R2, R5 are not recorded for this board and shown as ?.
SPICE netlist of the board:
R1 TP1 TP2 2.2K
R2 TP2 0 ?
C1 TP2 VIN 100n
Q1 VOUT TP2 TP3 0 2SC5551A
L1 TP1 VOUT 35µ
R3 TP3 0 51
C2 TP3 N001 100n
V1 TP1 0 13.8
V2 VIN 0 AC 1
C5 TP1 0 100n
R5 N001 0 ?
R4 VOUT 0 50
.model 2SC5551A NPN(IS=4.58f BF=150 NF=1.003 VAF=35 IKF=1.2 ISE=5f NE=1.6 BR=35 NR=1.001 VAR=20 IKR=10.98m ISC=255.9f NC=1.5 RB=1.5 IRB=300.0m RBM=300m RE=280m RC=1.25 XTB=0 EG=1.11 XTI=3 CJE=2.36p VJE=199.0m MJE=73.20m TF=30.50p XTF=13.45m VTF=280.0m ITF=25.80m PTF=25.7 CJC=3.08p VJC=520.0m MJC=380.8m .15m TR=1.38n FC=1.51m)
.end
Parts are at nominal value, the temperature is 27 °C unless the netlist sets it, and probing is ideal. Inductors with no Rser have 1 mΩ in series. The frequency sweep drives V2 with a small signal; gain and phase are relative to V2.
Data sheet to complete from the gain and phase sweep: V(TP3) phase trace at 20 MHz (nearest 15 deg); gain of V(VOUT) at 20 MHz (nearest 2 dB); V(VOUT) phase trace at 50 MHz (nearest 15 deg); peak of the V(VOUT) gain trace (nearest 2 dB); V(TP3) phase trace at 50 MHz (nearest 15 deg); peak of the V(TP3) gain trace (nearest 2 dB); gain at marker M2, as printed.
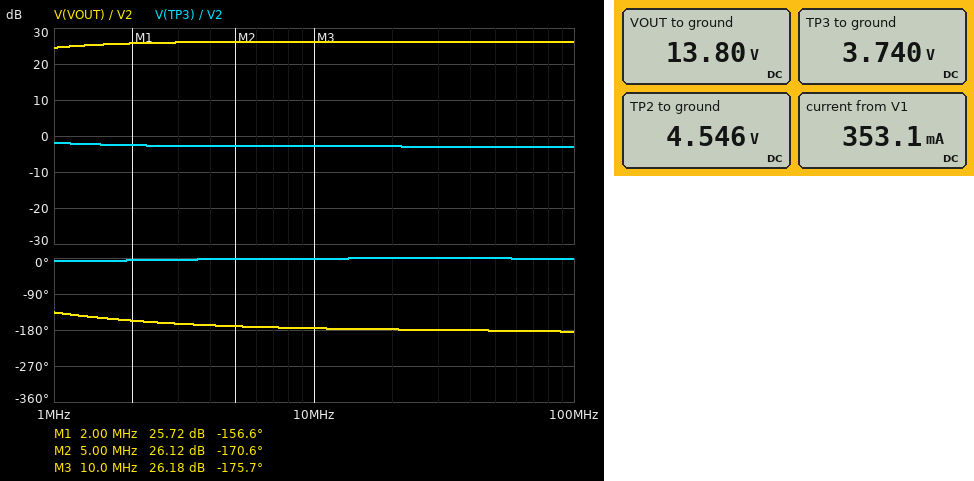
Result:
0 deg
26 dB
-180 deg
26 dB
0 deg
-2 dB
26.12 dB
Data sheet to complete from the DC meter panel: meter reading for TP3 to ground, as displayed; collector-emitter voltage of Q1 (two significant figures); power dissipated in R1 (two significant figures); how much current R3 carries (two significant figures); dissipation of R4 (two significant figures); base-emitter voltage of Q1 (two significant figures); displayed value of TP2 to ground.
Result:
3.740 V
10 V
39 mW
73 mA
3.8 W
810 mV
4.546 V
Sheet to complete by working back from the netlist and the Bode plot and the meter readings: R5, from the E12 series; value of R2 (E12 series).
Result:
1.8 Ω
1.2 kΩ
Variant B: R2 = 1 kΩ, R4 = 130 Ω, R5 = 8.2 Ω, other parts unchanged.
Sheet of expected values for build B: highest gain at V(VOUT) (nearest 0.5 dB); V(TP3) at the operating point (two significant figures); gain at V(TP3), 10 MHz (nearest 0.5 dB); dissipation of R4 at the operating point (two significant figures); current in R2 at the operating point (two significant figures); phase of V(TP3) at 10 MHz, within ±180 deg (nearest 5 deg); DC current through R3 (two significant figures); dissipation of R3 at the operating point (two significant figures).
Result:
24.5 dB
3.3 V
-1.0 dB
1.5 W
4.1 mA
0 deg
64 mA
210 mW
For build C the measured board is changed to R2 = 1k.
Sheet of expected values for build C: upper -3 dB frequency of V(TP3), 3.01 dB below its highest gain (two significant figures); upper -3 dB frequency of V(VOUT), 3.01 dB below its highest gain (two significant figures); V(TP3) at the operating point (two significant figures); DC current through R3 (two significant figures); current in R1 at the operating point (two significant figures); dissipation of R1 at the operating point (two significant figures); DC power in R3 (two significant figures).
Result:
290 MHz
1.6 GHz
3.3 V
64 mA
4.4 mA
43 mW
210 mW
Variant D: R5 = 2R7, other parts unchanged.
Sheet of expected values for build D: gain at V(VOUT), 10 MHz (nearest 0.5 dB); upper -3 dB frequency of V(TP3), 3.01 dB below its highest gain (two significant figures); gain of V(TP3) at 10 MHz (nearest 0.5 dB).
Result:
23.5 dB
1.2 GHz
-2.0 dB
